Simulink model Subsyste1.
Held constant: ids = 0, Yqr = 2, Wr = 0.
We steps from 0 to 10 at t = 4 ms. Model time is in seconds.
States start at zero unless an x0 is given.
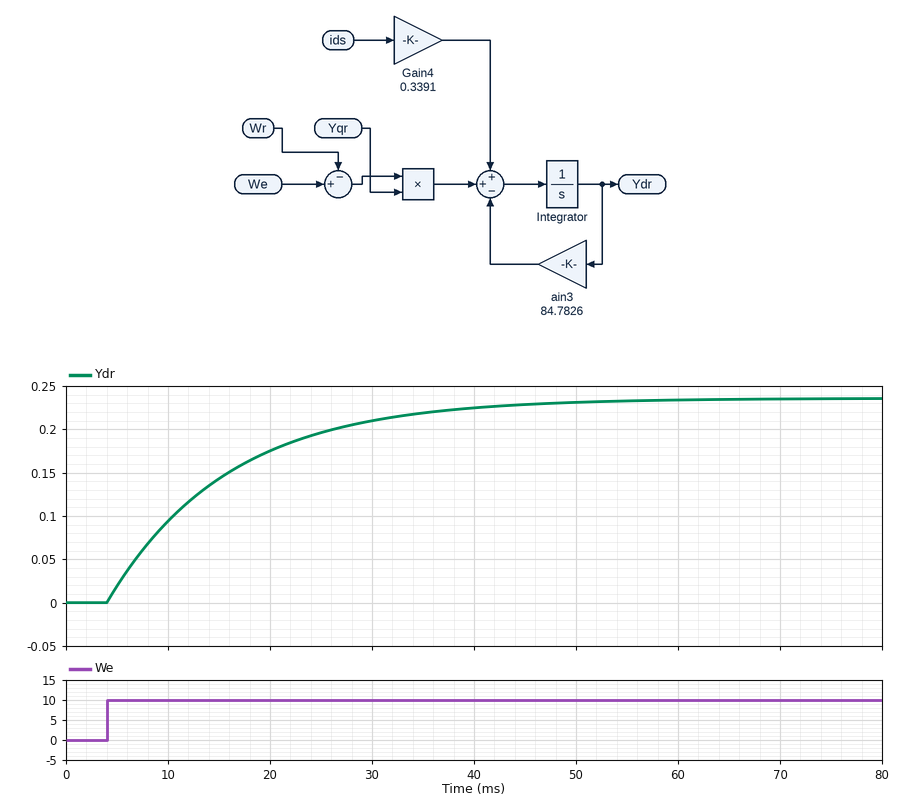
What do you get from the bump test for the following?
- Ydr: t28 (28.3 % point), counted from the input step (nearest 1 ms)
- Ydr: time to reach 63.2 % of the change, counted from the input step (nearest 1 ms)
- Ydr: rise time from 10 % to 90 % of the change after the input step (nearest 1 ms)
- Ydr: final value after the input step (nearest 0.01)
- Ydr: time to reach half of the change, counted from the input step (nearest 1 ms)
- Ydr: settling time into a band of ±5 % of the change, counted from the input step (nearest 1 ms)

4 ms
12 ms
26 ms
0.24
8 ms
35 ms
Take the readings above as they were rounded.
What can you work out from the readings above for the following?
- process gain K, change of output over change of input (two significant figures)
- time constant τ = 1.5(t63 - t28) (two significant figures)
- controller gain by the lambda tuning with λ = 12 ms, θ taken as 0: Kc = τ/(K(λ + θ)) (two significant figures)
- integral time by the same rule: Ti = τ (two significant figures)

0.024
12 ms
42
12 ms
